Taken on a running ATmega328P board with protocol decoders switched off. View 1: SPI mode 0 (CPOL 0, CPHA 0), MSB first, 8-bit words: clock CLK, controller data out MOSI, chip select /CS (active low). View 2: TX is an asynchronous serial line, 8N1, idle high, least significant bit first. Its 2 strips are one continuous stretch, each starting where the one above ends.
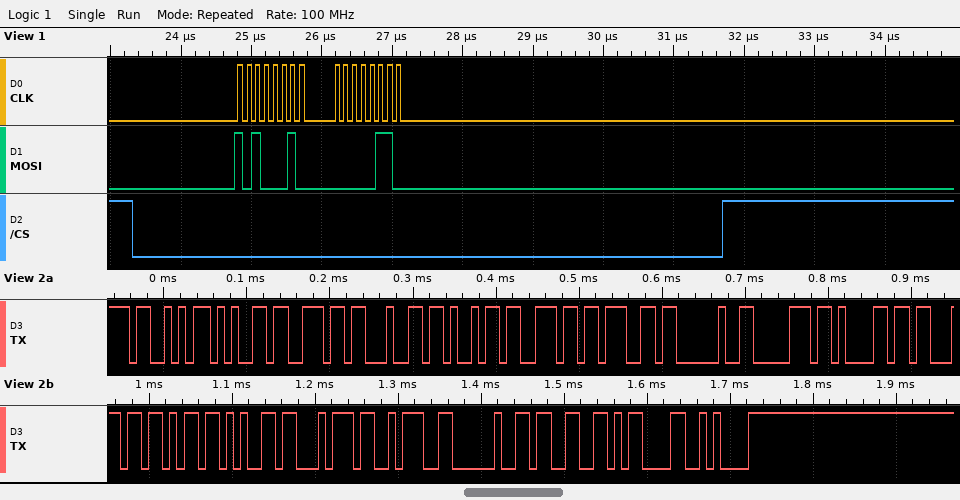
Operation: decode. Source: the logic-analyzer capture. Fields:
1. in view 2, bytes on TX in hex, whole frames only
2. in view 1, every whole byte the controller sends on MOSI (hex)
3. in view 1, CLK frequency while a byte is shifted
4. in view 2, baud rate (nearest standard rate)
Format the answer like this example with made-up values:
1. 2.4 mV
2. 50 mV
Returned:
1. 0x53 0x65 0x6E 0x64 0x69 0x6E 0x67 0x20 0x70 0x61 0x63 0x6B 0x65 0x74 0x3A 0x20 0x33 0x0D 0x0A
2. A2 06
3. 8 MHz
4. 115200 baud
